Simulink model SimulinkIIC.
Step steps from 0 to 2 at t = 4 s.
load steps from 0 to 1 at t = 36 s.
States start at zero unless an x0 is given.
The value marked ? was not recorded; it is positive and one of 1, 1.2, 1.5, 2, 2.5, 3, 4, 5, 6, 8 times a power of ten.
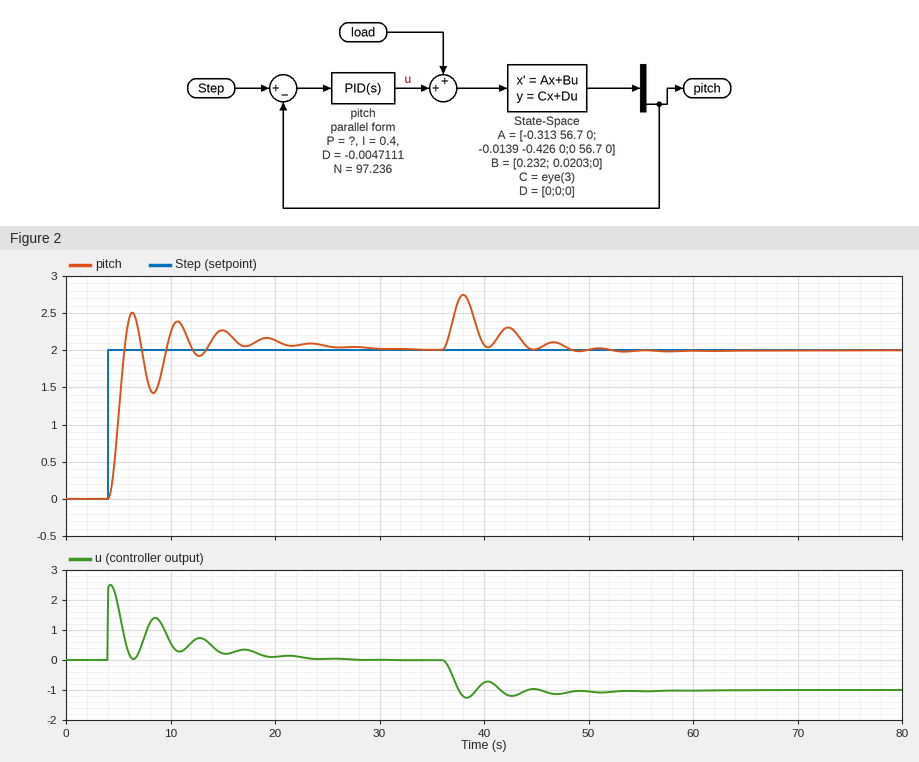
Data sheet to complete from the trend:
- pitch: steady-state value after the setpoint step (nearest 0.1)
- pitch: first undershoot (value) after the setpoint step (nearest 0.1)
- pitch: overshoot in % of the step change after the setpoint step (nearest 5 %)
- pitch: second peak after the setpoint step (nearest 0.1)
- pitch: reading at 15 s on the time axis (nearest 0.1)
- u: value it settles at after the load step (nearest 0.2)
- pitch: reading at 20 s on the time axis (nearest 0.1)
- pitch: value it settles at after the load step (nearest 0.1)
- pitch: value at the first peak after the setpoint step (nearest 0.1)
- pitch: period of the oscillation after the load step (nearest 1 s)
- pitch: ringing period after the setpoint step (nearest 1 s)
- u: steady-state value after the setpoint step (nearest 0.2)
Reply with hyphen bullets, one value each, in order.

- 2.0
- 1.4
- 25 %
- 2.4
- 2.3
- -1.0
- 2.1
- 2.0
- 2.5
- 4 s
- 4 s
- 0.0
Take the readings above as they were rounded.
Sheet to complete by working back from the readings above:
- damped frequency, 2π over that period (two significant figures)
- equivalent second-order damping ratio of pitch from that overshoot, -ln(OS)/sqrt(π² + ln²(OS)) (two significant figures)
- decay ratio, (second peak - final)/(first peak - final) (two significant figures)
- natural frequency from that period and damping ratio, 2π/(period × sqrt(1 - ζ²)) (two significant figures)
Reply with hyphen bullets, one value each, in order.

- 1.6 rad/s
- 0.40
- 0.80
- 1.7 rad/s
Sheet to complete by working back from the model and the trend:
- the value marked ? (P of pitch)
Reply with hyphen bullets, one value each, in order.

- 1.2
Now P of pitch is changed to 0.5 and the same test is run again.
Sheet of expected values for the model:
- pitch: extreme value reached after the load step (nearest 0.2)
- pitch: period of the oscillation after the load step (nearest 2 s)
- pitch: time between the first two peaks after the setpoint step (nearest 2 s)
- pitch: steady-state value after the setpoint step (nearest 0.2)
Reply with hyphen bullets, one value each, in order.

- 3.0
- 6 s
- 6 s
- 2.0
